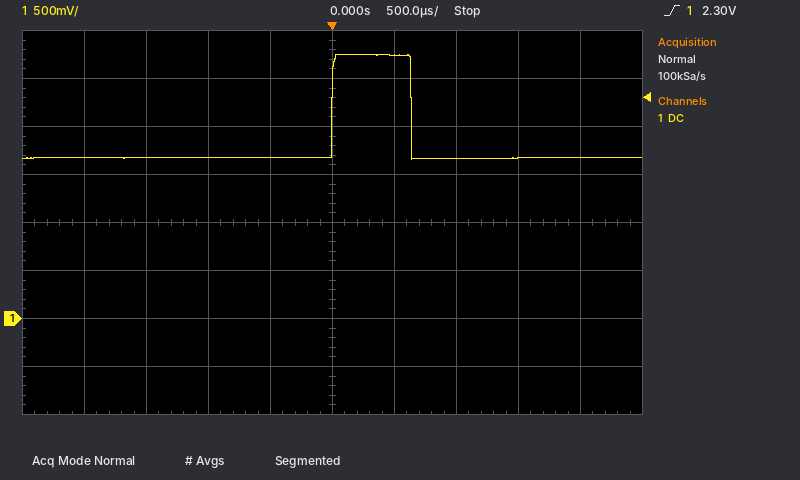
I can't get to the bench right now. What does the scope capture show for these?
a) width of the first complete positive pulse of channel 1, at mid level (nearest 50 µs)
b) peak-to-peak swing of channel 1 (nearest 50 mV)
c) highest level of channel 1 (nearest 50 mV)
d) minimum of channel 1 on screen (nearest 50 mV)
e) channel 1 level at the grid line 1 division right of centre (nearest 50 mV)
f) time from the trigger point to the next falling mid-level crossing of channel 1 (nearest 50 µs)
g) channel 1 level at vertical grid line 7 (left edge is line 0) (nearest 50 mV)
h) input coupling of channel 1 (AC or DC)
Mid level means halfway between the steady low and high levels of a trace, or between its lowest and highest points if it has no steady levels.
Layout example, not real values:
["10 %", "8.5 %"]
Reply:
["650 µs", "1.10 V", "2.75 V", "1.65 V", "2.75 V", "650 µs", "1.65 V", "DC"]
